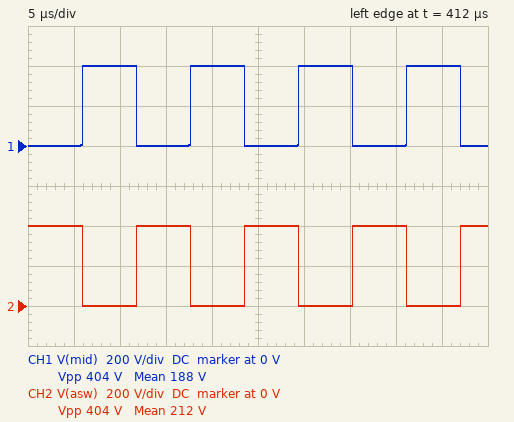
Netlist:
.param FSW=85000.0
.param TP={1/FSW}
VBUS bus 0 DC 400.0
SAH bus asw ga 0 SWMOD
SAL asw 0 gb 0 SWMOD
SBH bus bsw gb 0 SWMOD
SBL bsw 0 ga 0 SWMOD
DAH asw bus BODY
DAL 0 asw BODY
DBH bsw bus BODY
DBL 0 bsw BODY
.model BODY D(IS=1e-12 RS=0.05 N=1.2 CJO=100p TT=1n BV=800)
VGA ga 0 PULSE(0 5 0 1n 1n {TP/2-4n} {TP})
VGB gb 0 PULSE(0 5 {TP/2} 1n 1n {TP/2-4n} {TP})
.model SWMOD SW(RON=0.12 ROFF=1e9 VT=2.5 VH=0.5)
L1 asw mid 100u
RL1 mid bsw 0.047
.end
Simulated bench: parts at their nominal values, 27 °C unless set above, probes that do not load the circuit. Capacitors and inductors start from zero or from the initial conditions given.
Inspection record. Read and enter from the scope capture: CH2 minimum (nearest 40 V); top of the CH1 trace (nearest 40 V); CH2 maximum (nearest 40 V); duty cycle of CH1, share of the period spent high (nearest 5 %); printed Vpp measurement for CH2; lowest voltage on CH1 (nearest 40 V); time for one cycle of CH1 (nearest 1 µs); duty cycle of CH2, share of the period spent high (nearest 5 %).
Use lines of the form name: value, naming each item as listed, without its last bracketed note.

CH2 minimum: 0 V
top of the CH1 trace: 400 V
CH2 maximum: 400 V
duty cycle of CH1, share of the period spent high: 50 %
printed Vpp measurement for CH2: 404 V
lowest voltage on CH1: 0 V
time for one cycle of CH1: 12 µs
duty cycle of CH2, share of the period spent high: 50 %
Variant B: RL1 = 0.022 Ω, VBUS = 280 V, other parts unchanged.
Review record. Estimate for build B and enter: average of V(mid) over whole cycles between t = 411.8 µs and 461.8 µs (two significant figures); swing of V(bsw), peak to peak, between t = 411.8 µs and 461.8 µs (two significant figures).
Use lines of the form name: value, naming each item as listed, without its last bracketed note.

average of V(mid) over whole cycles between t = 411.8 µs and 461.8 µs: 140 V
swing of V(bsw), peak to peak, between t = 411.8 µs and 461.8 µs: 280 V
